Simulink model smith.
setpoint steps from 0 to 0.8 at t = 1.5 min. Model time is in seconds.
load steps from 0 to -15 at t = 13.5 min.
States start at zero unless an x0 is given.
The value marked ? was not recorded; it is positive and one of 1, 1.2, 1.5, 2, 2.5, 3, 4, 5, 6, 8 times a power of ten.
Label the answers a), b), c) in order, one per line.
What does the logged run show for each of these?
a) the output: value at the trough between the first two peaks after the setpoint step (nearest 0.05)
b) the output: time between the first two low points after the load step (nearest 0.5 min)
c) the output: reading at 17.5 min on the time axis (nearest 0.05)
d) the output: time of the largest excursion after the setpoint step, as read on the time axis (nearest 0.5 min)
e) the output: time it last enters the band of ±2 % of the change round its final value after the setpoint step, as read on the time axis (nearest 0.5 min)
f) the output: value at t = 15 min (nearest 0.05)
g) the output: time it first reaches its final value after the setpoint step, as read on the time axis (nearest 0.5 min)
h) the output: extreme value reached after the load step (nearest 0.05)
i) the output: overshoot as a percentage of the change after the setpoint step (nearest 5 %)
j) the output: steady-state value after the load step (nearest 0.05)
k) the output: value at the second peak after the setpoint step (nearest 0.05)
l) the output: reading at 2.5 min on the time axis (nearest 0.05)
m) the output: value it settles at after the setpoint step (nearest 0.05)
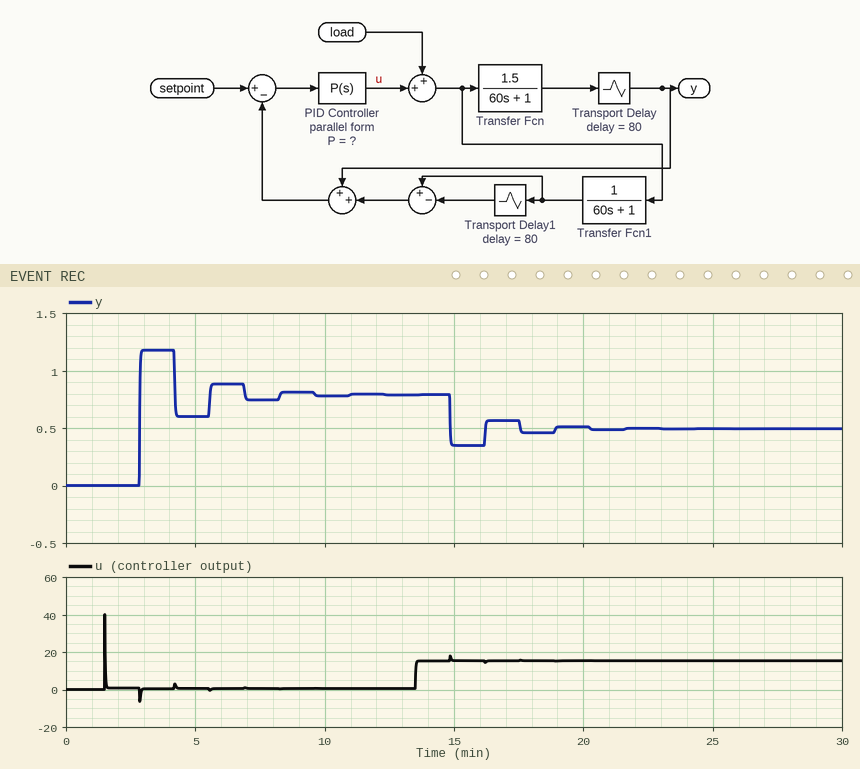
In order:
a) 0.60
b) 2.5 min
c) 0.55
d) 3.5 min
e) 9.5 min
f) 0.35
g) 3.0 min
h) 0.35
i) 50 %
j) 0.50
k) 0.90
l) 0.00
m) 0.80
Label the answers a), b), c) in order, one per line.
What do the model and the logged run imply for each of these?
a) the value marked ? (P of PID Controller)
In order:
a) 50
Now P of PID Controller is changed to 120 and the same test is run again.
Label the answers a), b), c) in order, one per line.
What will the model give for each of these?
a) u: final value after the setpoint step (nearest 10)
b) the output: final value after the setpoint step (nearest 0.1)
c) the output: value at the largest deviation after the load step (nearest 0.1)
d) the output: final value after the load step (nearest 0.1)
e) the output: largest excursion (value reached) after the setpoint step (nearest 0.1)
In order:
a) 0
b) 0.8
c) 0.6
d) 0.7
e) 1.2
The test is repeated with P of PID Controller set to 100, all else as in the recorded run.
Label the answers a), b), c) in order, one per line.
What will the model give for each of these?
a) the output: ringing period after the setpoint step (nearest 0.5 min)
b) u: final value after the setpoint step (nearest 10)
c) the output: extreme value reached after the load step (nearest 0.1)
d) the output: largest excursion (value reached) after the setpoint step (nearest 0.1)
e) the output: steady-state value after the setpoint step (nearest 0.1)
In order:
a) 2.5 min
b) 0
c) 0.6
d) 1.2
e) 0.8
